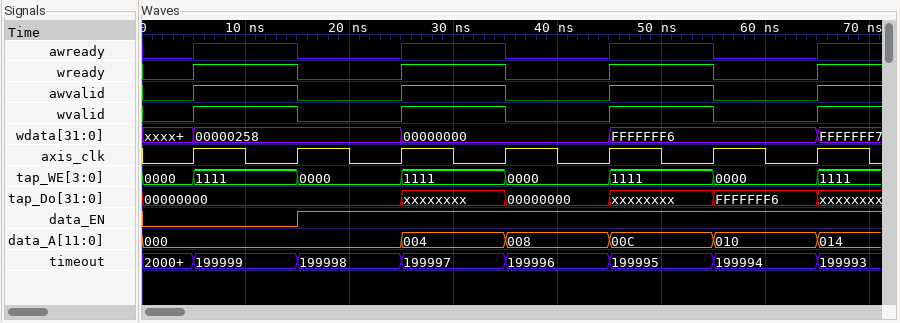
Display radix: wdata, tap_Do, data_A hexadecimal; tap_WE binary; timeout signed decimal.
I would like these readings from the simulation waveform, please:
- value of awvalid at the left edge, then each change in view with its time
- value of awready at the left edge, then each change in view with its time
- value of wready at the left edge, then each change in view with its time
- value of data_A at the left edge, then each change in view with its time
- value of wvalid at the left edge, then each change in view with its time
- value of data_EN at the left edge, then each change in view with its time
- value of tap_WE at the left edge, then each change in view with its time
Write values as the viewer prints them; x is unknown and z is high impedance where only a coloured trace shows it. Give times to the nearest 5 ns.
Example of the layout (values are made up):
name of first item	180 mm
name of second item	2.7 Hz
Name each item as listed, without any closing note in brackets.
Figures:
value of awvalid at the left edge, then each change in view with its time	0, 1 at 5 ns, 0 at 15 ns, 1 at 25 ns, 0 at 35 ns, 1 at 45 ns, 0 at 55 ns, 1 at 65 ns
value of awready at the left edge, then each change in view with its time	0, 1 at 5 ns, 0 at 15 ns, 1 at 25 ns, 0 at 35 ns, 1 at 45 ns, 0 at 55 ns, 1 at 65 ns
value of wready at the left edge, then each change in view with its time	0, 1 at 5 ns, 0 at 15 ns, 1 at 25 ns, 0 at 35 ns, 1 at 45 ns, 0 at 55 ns, 1 at 65 ns
value of data_A at the left edge, then each change in view with its time	000, 004 at 25 ns, 008 at 35 ns, 00C at 45 ns, 010 at 55 ns, 014 at 65 ns
value of wvalid at the left edge, then each change in view with its time	0, 1 at 5 ns, 0 at 15 ns, 1 at 25 ns, 0 at 35 ns, 1 at 45 ns, 0 at 55 ns, 1 at 65 ns
value of data_EN at the left edge, then each change in view with its time	0, 1 at 15 ns
value of tap_WE at the left edge, then each change in view with its time	0000, 1111 at 5 ns, 0000 at 15 ns, 1111 at 25 ns, 0000 at 35 ns, 1111 at 45 ns, 0000 at 55 ns, 1111 at 65 ns
